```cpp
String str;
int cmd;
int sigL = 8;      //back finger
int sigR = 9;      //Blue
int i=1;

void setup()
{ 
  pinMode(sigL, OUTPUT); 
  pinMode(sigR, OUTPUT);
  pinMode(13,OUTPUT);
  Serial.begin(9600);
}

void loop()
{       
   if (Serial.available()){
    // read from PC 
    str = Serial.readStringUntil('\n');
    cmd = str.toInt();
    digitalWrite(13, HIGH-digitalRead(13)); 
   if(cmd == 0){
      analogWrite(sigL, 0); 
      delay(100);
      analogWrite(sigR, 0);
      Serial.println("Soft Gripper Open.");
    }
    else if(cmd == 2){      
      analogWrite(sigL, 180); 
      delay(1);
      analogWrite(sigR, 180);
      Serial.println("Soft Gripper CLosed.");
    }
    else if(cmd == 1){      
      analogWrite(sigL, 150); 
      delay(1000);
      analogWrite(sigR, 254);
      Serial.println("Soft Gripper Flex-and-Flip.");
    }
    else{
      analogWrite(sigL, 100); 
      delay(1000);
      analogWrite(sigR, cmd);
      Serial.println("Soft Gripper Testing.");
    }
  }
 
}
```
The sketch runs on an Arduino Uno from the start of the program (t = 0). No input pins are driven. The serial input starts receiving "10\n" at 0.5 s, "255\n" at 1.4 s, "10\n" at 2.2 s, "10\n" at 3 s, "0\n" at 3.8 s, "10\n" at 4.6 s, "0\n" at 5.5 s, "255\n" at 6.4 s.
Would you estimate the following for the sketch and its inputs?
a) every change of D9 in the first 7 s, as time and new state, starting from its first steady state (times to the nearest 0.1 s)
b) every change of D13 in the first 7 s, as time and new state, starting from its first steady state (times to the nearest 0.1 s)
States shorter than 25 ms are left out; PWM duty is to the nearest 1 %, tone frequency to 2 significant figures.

0 s low; 1.5 s PWM 4 %; 2.5 s high; 3.5 s PWM 4 %; 4.6 s low; 5.6 s PWM 4 %; 5.7 s low
0 s low; 0.5 s high; 1.5 s low; 2.5 s high; 3.5 s low; 4.5 s high; 4.6 s low; 5.6 s high; 6.4 s low
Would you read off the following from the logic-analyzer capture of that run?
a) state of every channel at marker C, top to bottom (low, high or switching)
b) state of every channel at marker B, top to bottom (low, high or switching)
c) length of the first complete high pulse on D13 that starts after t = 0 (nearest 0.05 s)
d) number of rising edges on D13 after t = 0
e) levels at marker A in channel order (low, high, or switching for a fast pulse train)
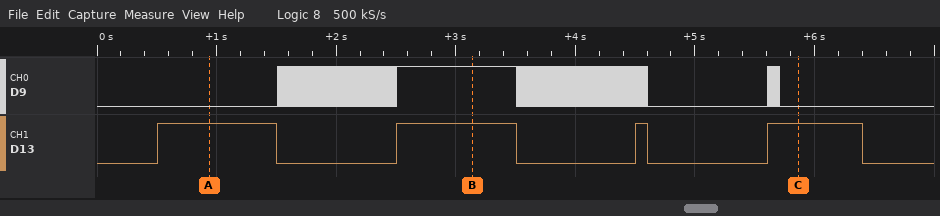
D9 low, D13 high
D9 high, D13 high
1.00 s
4
D9 low, D13 high
